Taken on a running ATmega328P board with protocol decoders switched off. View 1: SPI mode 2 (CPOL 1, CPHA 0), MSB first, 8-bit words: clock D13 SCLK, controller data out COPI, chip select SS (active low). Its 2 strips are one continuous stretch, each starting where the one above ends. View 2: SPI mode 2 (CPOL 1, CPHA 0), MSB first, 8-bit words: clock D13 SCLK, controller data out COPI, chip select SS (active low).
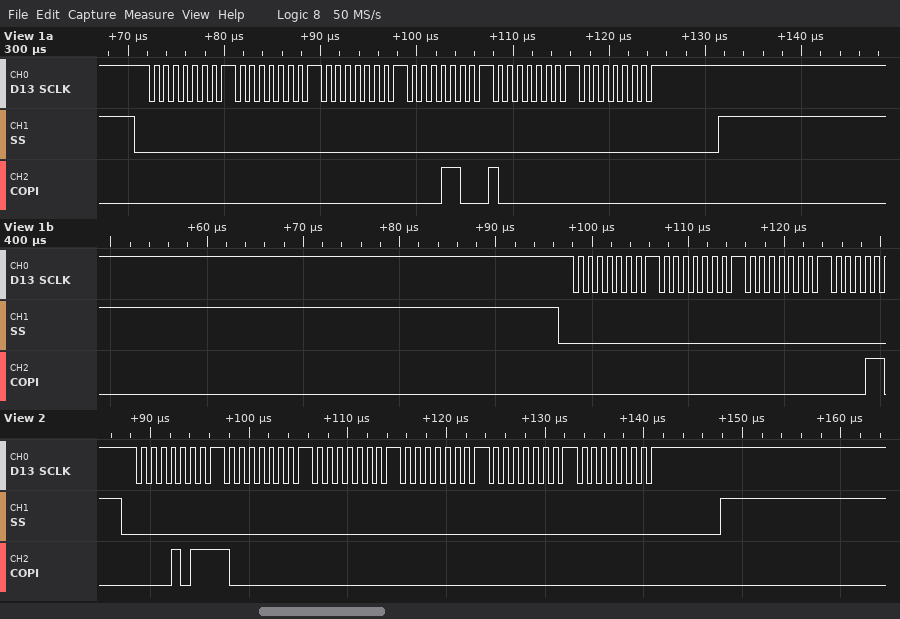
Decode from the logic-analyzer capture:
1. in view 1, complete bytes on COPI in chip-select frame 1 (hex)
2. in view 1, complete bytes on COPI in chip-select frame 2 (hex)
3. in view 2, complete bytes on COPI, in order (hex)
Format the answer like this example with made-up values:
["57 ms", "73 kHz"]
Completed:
["00 00 00 0C 80 00", "00 00 00", "0x0B 0x80 0x00 0x00 0x00 0x00"]
